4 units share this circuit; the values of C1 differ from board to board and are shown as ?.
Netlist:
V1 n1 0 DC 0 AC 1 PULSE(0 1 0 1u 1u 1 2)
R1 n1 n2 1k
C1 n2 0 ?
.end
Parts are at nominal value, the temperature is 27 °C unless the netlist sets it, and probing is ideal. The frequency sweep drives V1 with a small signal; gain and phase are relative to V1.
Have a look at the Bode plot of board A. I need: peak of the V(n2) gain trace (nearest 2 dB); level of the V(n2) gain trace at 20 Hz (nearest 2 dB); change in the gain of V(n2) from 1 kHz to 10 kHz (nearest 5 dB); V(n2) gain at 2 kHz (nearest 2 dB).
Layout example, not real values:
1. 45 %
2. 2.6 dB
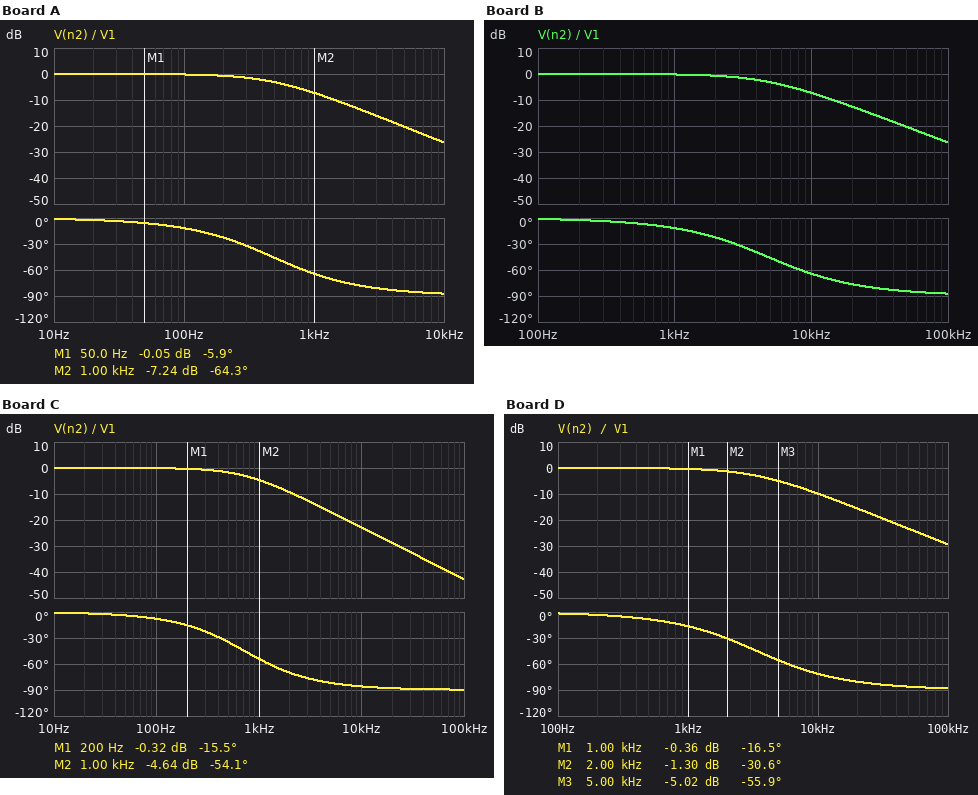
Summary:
1. 0 dB
2. 0 dB
3. -20 dB
4. -12 dB
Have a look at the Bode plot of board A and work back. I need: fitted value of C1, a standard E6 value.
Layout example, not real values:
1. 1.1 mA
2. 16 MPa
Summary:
1. 330 nF
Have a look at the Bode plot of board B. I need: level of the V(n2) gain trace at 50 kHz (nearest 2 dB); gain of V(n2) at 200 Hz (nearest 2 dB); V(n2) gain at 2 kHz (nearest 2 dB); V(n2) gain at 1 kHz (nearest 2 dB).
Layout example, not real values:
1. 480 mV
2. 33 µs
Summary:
1. -20 dB
2. 0 dB
3. 0 dB
4. 0 dB
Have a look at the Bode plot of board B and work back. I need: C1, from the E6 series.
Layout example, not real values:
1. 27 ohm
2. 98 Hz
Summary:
1. 33 nF
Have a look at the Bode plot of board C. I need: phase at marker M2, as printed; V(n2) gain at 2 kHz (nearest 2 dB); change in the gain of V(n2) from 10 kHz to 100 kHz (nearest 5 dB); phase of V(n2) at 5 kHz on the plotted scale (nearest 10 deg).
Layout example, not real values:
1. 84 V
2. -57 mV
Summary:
1. -54.1 deg
2. -10 dB
3. -20 dB
4. -80 deg
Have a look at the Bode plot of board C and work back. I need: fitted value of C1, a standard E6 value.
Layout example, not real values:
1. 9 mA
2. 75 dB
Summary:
1. 220 nF
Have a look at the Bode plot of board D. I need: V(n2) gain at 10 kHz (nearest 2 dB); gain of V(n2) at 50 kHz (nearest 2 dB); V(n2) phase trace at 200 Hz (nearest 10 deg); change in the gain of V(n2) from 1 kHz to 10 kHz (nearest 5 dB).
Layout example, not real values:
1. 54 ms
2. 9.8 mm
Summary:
1. -10 dB
2. -24 dB
3. 0 deg
4. -10 dB
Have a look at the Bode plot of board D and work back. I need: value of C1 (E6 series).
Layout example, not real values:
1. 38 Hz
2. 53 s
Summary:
1. 47 nF
